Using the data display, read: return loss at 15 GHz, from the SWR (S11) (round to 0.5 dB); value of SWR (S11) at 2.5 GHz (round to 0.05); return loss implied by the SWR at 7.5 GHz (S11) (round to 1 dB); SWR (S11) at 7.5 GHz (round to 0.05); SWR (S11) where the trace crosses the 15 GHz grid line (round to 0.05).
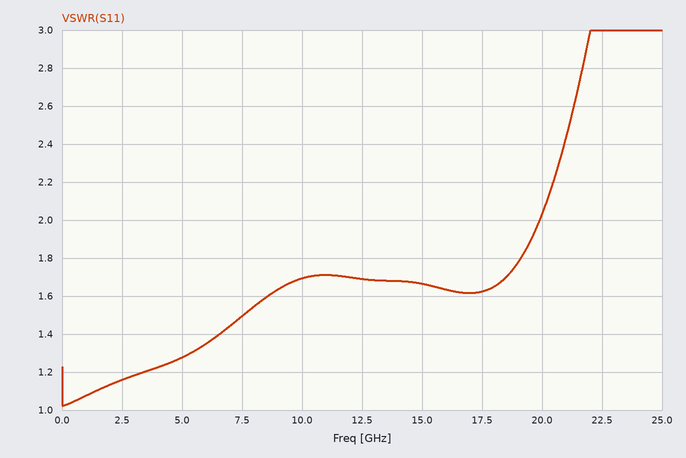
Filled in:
12.0 dB
1.15
14 dB
1.50
1.65
